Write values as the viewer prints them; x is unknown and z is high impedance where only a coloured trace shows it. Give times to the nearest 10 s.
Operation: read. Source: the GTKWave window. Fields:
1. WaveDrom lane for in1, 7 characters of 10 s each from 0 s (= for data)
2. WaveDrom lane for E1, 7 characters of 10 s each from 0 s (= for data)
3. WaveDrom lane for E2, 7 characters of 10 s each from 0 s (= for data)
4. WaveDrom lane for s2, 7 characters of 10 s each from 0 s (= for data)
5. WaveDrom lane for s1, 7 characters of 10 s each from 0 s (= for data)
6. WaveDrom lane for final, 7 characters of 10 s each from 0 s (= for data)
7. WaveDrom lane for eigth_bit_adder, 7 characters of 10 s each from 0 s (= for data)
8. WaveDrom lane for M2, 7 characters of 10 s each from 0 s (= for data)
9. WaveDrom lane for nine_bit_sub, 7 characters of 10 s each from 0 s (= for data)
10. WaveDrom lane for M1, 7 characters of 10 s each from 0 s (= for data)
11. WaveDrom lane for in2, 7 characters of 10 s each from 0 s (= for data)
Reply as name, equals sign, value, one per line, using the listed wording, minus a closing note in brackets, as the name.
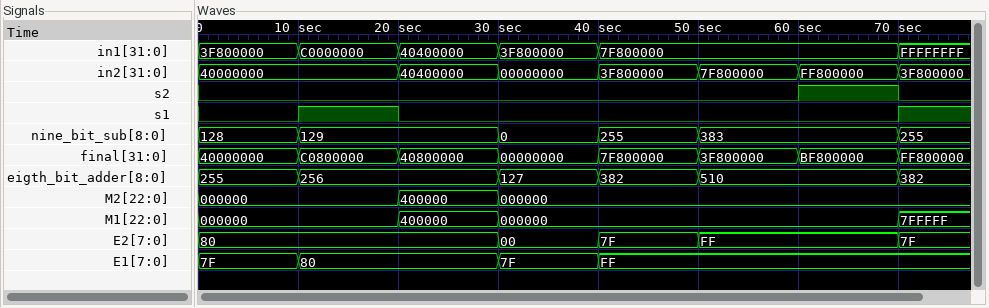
WaveDrom lane for in1, 7 characters of 10 s each from 0 s = {name: 'in1', wave: '=====..', data: '3F800000 C0000000 40400000 3F800000 7F800000'}
WaveDrom lane for E1, 7 characters of 10 s each from 0 s = {name: 'E1', wave: '==.==..', data: '7F 80 7F FF'}
WaveDrom lane for E2, 7 characters of 10 s each from 0 s = {name: 'E2', wave: '=..===.', data: '80 00 7F FF'}
WaveDrom lane for s2, 7 characters of 10 s each from 0 s = {name: 's2', wave: '0.....1'}
WaveDrom lane for s1, 7 characters of 10 s each from 0 s = {name: 's1', wave: '010....'}
WaveDrom lane for final, 7 characters of 10 s each from 0 s = {name: 'final', wave: '=======', data: '40000000 C0800000 40800000 00000000 7F800000 3F800000 BF800000'}
WaveDrom lane for eigth_bit_adder, 7 characters of 10 s each from 0 s = {name: 'eigth_bit_adder', wave: '==.===.', data: '255 256 127 382 510'}
WaveDrom lane for M2, 7 characters of 10 s each from 0 s = {name: 'M2', wave: '=.==...', data: '000000 400000 000000'}
WaveDrom lane for nine_bit_sub, 7 characters of 10 s each from 0 s = {name: 'nine_bit_sub', wave: '==.===.', data: '128 129 0 255 383'}
WaveDrom lane for M1, 7 characters of 10 s each from 0 s = {name: 'M1', wave: '=.==...', data: '000000 400000 000000'}
WaveDrom lane for in2, 7 characters of 10 s each from 0 s = {name: 'in2', wave: '=.=====', data: '40000000 40400000 00000000 3F800000 7F800000 FF800000'}
